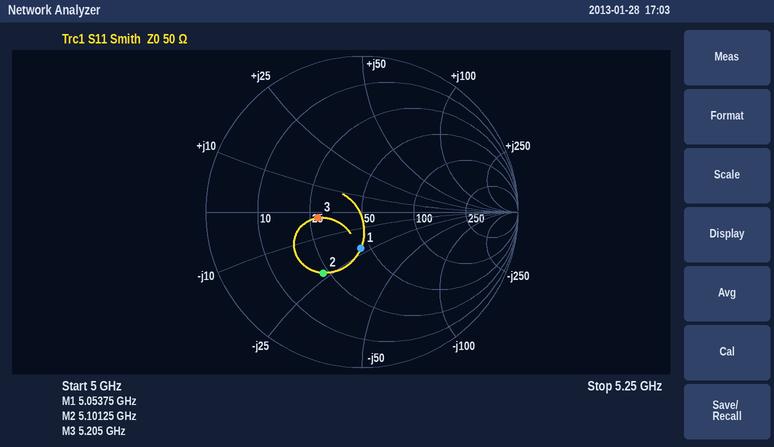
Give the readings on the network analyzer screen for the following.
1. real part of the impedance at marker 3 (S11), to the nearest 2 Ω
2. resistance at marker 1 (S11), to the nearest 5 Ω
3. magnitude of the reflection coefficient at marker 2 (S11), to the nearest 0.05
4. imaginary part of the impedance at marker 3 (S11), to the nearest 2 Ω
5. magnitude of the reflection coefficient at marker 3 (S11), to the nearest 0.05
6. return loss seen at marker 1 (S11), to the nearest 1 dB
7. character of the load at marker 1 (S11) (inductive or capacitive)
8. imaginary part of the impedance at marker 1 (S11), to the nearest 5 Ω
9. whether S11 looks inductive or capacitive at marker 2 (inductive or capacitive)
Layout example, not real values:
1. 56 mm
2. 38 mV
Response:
1. 28 Ω
2. 45 Ω
3. 0.45
4. -2 Ω
5. 0.30
6. 13 dB
7. capacitive
8. -20 Ω
9. capacitive
